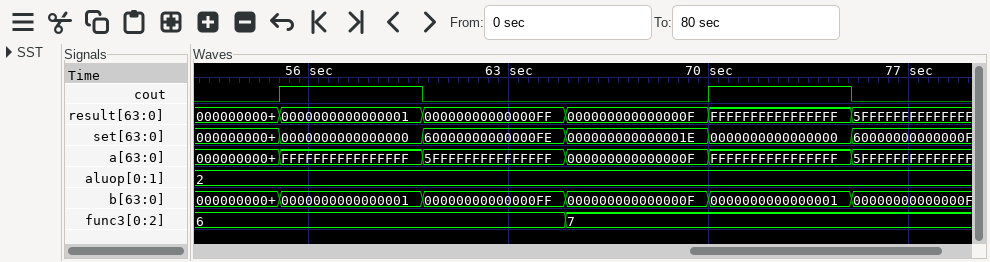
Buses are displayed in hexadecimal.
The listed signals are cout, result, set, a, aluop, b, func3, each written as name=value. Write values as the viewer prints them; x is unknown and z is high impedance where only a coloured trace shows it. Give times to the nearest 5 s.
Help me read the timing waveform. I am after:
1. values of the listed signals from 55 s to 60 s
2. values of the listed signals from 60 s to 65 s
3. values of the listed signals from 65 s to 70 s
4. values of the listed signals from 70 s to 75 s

cout=1, result=0000000000000001, set=0000000000000000, a=FFFFFFFFFFFFFFFF, aluop=2, b=0000000000000001, func3=6
cout=0, result=00000000000000FF, set=60000000000000FE, a=5FFFFFFFFFFFFFFF, aluop=2, b=00000000000000FF, func3=6
cout=0, result=000000000000000F, set=000000000000001E, a=000000000000000F, aluop=2, b=000000000000000F, func3=7
cout=1, result=FFFFFFFFFFFFFFFF, set=0000000000000000, a=FFFFFFFFFFFFFFFF, aluop=2, b=0000000000000001, func3=7
